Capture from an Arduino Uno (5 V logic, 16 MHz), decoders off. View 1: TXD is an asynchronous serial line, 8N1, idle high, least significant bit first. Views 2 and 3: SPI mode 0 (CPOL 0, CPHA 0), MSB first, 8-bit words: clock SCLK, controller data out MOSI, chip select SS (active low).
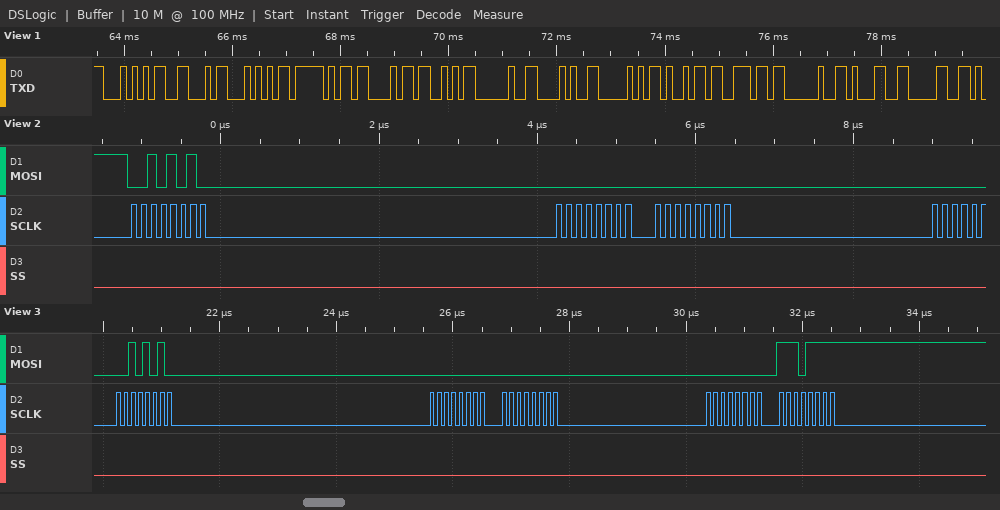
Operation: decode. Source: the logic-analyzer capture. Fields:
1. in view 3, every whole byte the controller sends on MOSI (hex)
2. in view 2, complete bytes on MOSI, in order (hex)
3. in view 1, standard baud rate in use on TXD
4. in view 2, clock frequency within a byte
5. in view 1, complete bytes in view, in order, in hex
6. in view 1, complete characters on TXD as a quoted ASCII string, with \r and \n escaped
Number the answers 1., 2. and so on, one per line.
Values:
1. 0x2A 0x00 0x00 0x00 0xEF
2. 2A 00 00
3. 9600 baud
4. 8 MHz
5. 54 46 54 5F 43 53 20 28 50 69 6E 20 31 30
6. "TFT_CS (Pin 10"
